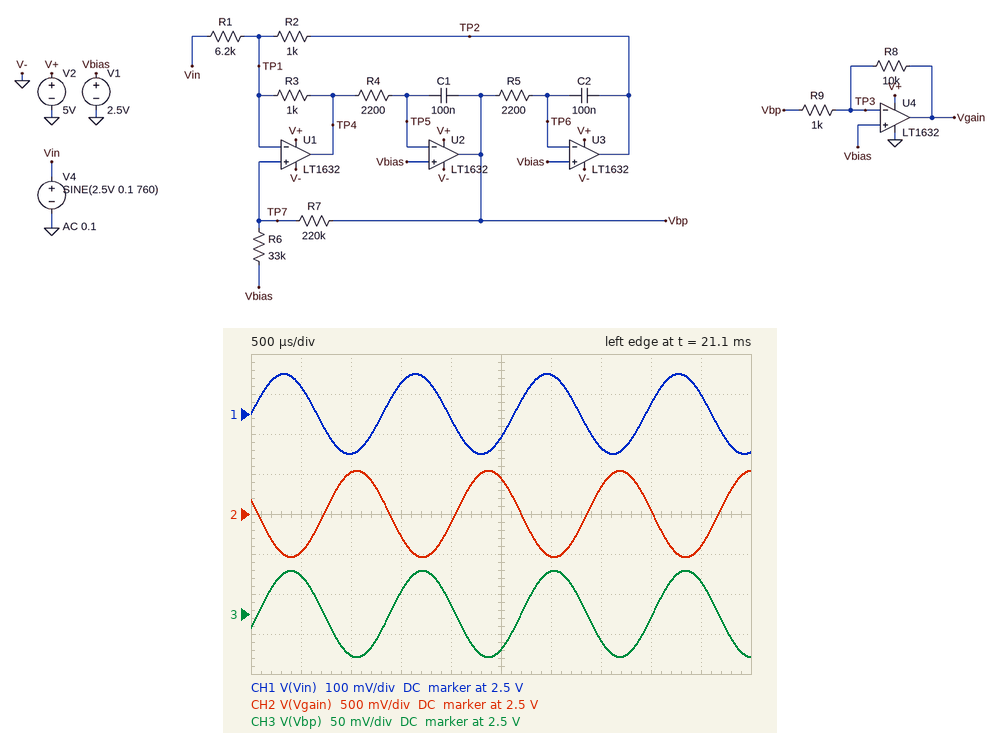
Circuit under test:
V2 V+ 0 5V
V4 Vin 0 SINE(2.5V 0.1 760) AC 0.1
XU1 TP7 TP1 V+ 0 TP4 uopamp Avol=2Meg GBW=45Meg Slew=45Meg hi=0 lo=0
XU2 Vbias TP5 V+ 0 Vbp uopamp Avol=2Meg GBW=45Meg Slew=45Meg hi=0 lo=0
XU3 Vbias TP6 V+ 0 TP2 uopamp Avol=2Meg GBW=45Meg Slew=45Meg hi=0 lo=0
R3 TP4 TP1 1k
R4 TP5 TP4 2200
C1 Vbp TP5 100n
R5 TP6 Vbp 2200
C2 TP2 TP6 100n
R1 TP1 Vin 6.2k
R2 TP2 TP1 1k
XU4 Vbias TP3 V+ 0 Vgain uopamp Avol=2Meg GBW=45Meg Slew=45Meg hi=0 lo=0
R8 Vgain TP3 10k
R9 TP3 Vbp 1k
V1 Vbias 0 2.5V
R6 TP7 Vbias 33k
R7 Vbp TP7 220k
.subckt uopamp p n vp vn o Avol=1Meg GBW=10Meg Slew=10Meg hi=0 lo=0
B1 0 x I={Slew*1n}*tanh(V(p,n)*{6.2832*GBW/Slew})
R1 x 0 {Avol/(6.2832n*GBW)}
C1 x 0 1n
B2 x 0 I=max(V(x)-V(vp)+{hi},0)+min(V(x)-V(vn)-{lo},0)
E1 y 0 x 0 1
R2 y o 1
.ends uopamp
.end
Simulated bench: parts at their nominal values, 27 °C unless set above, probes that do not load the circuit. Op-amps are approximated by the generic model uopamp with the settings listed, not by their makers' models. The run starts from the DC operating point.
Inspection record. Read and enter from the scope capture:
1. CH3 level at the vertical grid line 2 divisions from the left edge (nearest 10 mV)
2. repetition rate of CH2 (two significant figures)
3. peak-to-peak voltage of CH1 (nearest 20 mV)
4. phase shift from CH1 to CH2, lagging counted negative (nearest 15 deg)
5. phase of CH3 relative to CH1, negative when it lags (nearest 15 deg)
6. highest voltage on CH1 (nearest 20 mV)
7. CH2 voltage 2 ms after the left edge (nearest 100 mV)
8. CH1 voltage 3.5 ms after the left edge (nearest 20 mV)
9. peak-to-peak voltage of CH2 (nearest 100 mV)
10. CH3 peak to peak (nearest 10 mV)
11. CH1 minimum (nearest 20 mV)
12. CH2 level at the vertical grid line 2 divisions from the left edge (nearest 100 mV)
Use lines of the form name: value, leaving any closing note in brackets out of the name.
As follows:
CH3 level at the vertical grid line 2 divisions from the left edge: 2.45 V
repetition rate of CH2: 760 Hz
peak-to-peak voltage of CH1: 200 mV
phase shift from CH1 to CH2, lagging counted negative: 165 deg
phase of CH3 relative to CH1, negative when it lags: -15 deg
highest voltage on CH1: 2.60 V
CH2 voltage 2 ms after the left edge: 2.4 V
CH1 voltage 3.5 ms after the left edge: 2.42 V
peak-to-peak voltage of CH2: 1.1 V
CH3 peak to peak: 110 mV
CH1 minimum: 2.40 V
CH2 level at the vertical grid line 2 divisions from the left edge: 3.0 V
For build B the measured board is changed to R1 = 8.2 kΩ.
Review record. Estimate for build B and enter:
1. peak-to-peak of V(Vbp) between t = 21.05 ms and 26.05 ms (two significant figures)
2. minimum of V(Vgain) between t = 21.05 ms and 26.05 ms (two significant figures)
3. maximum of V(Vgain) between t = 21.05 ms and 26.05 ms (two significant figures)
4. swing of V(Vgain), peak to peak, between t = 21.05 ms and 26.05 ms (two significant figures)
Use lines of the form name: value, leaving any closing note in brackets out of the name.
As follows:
peak-to-peak of V(Vbp) between t = 21.05 ms and 26.05 ms: 83 mV
minimum of V(Vgain) between t = 21.05 ms and 26.05 ms: 2.1 V
maximum of V(Vgain) between t = 21.05 ms and 26.05 ms: 2.9 V
swing of V(Vgain), peak to peak, between t = 21.05 ms and 26.05 ms: 830 mV
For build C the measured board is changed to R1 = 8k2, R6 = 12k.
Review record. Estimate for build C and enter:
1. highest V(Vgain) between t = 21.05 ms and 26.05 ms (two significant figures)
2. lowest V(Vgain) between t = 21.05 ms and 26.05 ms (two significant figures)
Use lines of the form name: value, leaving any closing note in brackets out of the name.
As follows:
highest V(Vgain) between t = 21.05 ms and 26.05 ms: 3.3 V
lowest V(Vgain) between t = 21.05 ms and 26.05 ms: 1.7 V
